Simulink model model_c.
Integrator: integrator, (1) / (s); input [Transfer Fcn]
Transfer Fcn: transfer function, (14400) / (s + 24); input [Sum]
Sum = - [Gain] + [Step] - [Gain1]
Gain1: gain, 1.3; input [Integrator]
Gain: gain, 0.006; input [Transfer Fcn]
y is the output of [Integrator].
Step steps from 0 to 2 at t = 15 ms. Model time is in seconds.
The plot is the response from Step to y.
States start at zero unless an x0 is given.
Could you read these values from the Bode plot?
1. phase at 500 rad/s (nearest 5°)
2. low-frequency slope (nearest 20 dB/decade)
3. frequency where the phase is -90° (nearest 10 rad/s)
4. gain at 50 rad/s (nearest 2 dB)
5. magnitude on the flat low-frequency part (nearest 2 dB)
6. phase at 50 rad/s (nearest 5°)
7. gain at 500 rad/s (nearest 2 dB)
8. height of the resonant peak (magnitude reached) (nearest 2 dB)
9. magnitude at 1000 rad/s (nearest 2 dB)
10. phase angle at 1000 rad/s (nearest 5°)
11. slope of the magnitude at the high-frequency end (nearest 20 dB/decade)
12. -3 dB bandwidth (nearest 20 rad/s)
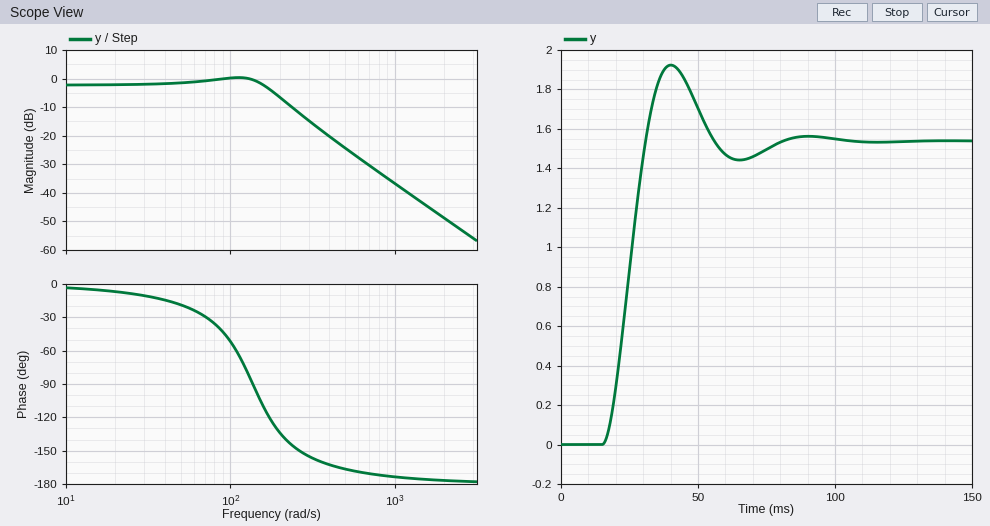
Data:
-165°
0 dB/decade
140 rad/s
-2 dB
-2 dB
-20°
-24 dB
0 dB
-36 dB
-175°
-40 dB/decade
180 rad/s
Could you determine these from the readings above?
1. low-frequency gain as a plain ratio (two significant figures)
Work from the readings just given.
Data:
0.79
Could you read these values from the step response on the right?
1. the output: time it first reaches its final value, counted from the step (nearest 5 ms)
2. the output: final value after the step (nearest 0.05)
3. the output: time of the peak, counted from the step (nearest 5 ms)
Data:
15 ms
1.55
25 ms
